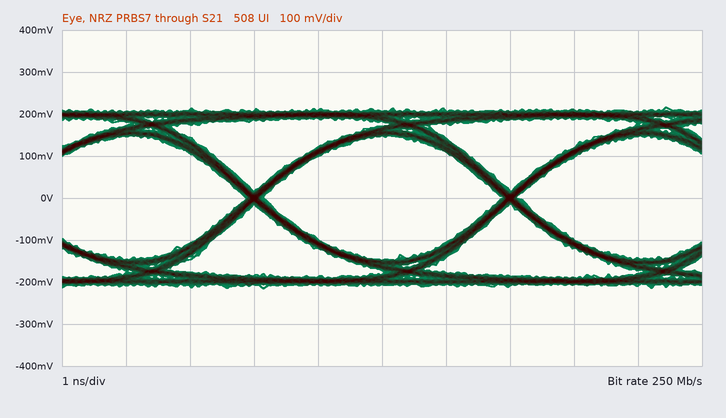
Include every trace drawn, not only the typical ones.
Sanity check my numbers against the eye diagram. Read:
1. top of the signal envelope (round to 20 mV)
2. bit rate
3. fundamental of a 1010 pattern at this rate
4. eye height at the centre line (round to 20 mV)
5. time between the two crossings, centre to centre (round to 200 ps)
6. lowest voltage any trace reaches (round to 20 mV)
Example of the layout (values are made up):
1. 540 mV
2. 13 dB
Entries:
1. 220 mV
2. 250 Mb/s
3. 125 MHz
4. 300 mV
5. 4.0 ns
6. -220 mV
